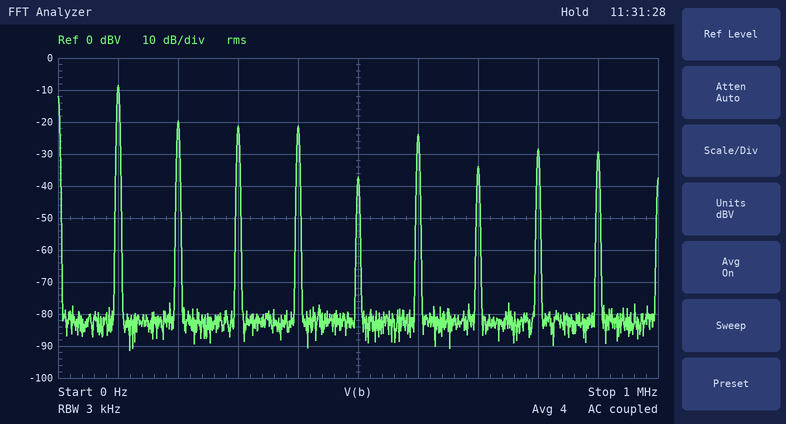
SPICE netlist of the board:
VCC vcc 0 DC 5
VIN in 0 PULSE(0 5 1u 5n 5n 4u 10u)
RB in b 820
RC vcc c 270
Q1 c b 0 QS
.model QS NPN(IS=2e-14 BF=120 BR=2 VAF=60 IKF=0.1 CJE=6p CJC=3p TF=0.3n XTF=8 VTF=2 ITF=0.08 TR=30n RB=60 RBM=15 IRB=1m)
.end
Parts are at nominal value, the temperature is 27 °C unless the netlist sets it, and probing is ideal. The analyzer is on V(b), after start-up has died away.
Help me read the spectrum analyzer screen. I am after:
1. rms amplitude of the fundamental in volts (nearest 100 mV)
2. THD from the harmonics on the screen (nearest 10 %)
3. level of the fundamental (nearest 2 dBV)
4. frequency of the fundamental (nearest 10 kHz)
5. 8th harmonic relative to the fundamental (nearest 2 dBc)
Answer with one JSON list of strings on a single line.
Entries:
["400 mV", "50 %", "-8 dBV", "100 kHz", "-20 dBc"]
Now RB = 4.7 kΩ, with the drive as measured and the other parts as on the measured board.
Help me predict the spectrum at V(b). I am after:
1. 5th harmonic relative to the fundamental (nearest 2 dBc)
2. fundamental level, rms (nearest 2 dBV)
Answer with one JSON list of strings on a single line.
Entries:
["-24 dBc", "-10 dBV"]
